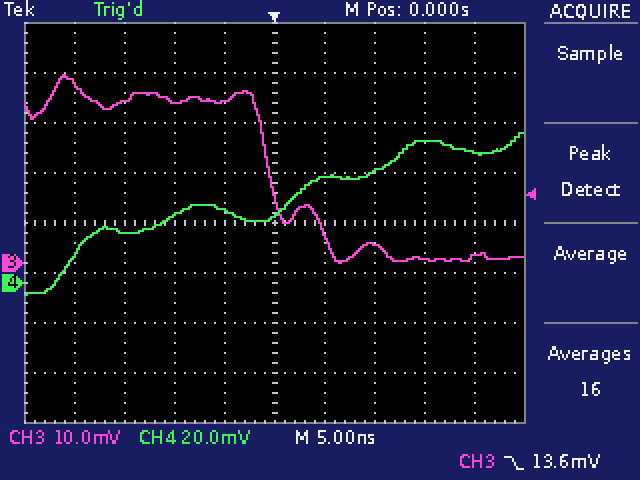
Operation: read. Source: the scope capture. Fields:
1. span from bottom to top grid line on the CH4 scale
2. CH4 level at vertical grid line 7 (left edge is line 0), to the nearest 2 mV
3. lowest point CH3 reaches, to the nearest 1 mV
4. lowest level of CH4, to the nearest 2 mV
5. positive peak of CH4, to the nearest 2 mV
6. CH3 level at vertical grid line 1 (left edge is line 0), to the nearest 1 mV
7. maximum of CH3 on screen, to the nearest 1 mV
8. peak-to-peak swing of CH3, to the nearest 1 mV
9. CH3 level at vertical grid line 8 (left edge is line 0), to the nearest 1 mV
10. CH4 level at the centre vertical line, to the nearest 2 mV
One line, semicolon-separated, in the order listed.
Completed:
160 mV; 44 mV; 0 mV; -4 mV; 60 mV; 36 mV; 38 mV; 38 mV; 1 mV; 26 mV
